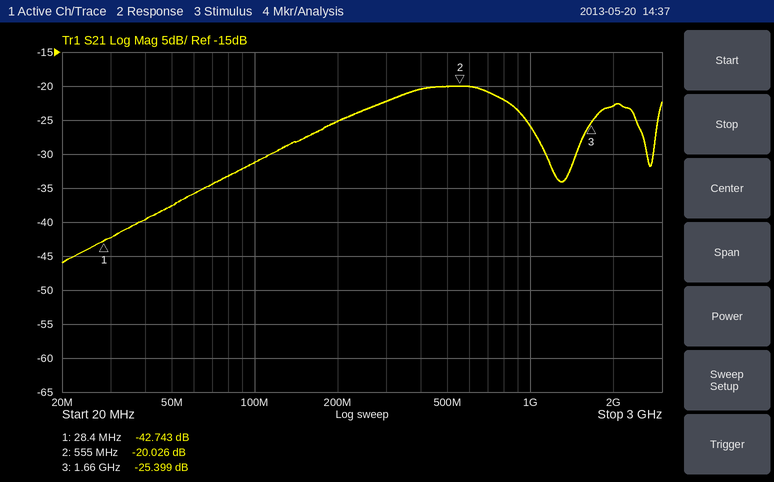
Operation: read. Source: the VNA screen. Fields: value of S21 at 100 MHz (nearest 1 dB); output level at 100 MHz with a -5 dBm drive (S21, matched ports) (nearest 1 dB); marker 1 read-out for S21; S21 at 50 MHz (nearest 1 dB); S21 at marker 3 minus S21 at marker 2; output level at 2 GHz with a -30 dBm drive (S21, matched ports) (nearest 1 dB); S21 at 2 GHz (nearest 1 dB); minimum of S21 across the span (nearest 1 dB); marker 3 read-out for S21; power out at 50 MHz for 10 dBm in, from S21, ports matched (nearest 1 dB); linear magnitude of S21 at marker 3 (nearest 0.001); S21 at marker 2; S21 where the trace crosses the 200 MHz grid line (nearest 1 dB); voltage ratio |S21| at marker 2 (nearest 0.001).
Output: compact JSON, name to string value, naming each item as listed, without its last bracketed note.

{"value of S21 at 100 MHz": "-31 dB", "output level at 100 MHz with a -5 dBm drive (S21, matched ports)": "-36 dBm", "marker 1 read-out for S21": "-42.743 dB", "S21 at 50 MHz": "-38 dB", "S21 at marker 3 minus S21 at marker 2": "-5.373 dB", "output level at 2 GHz with a -30 dBm drive (S21, matched ports)": "-53 dBm", "S21 at 2 GHz": "-23 dB", "minimum of S21 across the span": "-46 dB", "marker 3 read-out for S21": "-25.399 dB", "power out at 50 MHz for 10 dBm in, from S21, ports matched": "-28 dBm", "linear magnitude of S21 at marker 3": "0.054", "S21 at marker 2": "-20.026 dB", "S21 where the trace crosses the 200 MHz grid line": "-25 dB", "voltage ratio |S21| at marker 2": "0.100"}
